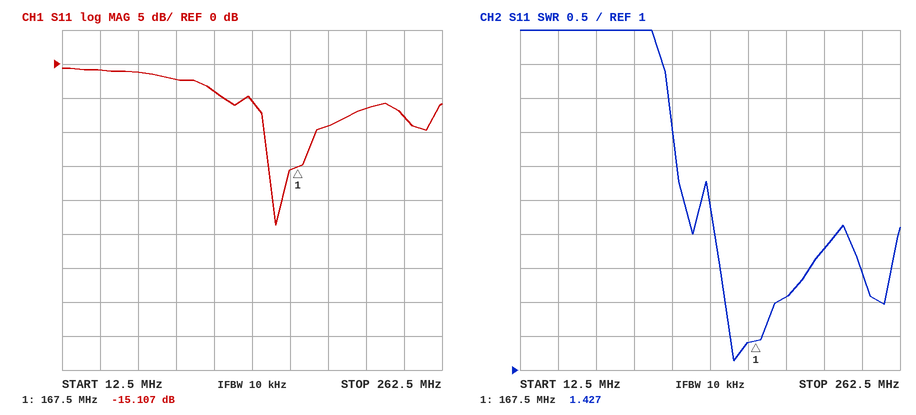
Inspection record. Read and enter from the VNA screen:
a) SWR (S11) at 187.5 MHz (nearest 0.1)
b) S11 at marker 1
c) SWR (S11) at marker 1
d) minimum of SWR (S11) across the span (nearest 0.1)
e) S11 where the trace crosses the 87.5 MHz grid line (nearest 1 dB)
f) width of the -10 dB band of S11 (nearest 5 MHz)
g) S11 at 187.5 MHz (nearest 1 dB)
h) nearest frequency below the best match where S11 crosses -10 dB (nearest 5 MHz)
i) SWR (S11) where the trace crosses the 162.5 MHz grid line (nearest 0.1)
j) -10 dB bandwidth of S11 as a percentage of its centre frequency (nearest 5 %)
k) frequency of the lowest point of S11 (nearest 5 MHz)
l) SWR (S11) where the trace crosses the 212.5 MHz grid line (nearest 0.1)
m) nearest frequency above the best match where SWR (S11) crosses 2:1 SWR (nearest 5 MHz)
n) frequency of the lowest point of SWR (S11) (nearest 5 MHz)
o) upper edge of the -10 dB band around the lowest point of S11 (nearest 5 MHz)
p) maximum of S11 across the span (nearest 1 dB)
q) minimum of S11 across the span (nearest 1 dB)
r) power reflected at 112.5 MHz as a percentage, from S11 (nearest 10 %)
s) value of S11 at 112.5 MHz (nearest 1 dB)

2.1
-15.107 dB
1.427
1.1
-2 dB
35 MHz
-9 dB
145 MHz
1.4
20 %
155 MHz
2.8
180 MHz
155 MHz
180 MHz
-1 dB
-24 dB
40 %
-4 dB
